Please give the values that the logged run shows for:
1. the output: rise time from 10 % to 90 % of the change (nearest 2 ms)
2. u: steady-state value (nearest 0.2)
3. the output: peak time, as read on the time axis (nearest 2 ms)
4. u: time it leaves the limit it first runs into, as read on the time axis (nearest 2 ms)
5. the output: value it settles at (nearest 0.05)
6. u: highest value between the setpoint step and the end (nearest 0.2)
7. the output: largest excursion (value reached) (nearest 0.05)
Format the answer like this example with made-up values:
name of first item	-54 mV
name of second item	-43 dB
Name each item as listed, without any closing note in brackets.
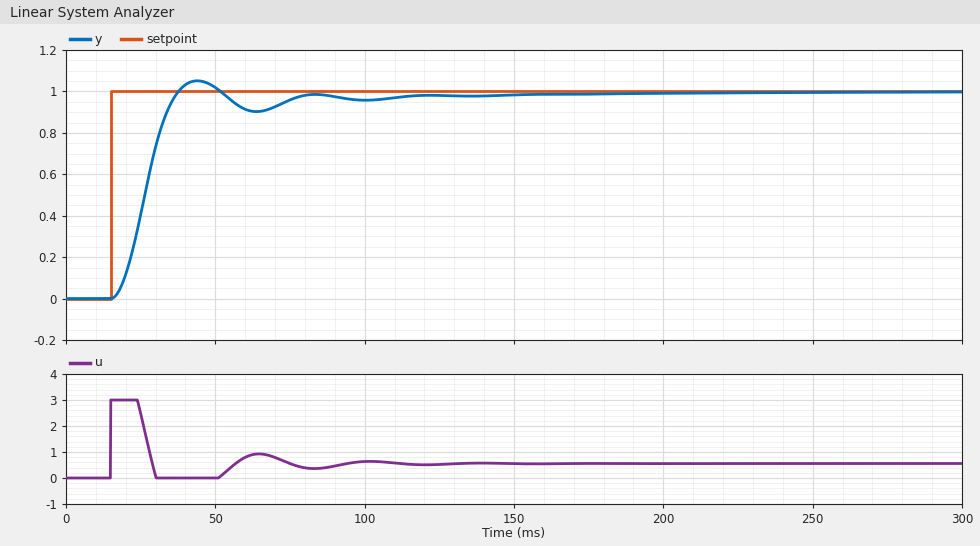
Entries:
the output: rise time from 10 % to 90 % of the change	14 ms
u: steady-state value	0.6
the output: peak time, as read on the time axis	44 ms
u: time it leaves the limit it first runs into, as read on the time axis	24 ms
the output: value it settles at	1.00
u: highest value between the setpoint step and the end	3.0
the output: largest excursion (value reached)	1.05
